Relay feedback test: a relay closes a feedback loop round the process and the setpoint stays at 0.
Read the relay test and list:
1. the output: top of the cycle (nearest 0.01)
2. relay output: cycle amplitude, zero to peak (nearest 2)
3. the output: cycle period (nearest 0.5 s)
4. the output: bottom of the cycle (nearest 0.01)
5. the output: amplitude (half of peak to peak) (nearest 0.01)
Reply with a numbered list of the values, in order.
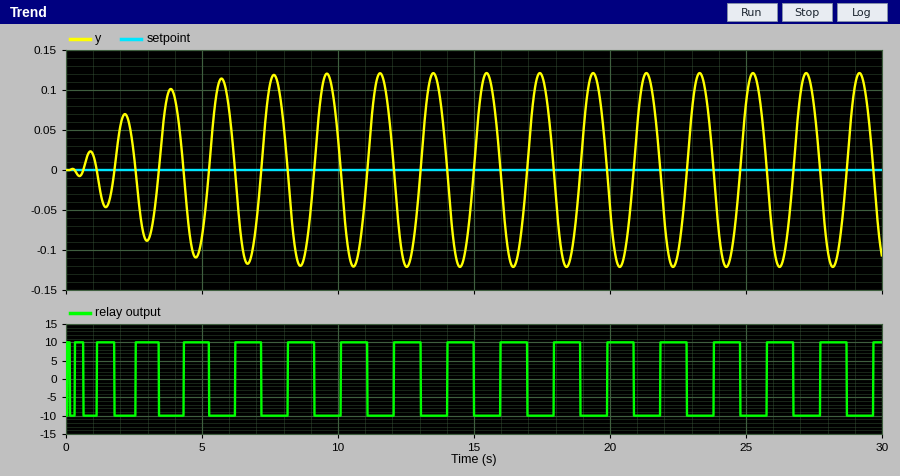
1. 0.12
2. 10
3. 2.0 s
4. -0.12
5. 0.12
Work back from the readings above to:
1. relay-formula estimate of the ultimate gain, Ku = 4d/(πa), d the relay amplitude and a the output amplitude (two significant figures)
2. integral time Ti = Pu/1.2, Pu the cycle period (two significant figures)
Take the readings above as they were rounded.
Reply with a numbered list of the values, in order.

1. 110
2. 1.7 s
